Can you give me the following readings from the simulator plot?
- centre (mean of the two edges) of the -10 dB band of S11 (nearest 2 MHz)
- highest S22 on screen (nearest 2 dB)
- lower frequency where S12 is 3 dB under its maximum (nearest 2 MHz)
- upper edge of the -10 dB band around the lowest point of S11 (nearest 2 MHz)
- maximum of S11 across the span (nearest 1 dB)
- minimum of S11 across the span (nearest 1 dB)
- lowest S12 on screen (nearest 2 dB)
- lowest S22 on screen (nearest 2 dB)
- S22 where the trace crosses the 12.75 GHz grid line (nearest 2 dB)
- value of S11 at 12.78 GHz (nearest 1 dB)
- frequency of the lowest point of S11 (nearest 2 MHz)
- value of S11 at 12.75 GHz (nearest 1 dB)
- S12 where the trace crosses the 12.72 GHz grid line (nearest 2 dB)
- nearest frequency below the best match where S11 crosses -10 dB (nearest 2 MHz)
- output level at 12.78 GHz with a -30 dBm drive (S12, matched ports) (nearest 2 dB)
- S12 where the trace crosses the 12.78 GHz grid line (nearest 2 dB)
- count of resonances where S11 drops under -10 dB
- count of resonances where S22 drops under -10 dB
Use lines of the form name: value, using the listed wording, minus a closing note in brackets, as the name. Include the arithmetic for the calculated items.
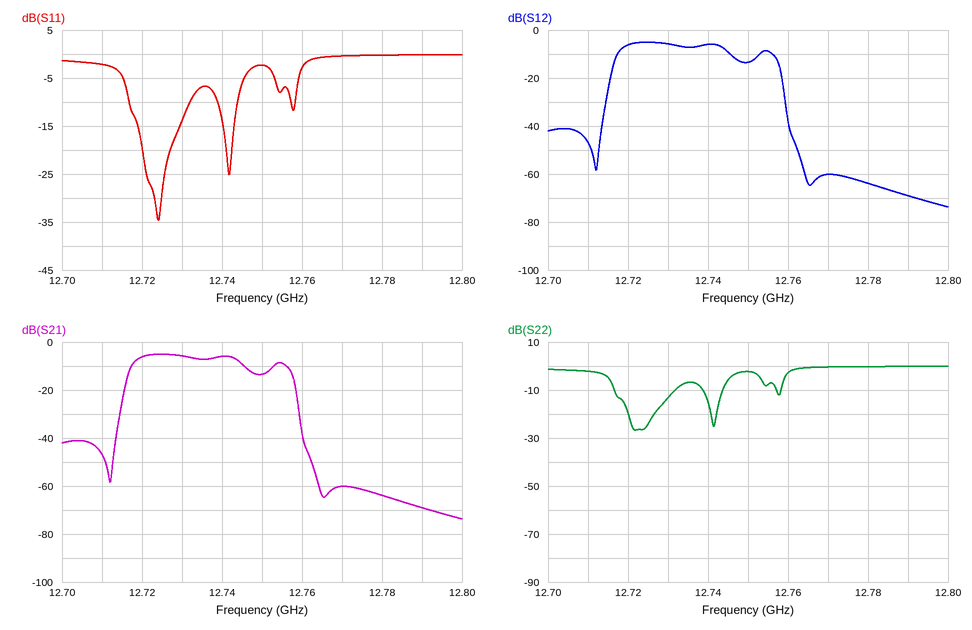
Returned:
centre (mean of the two edges) of the -10 dB band of S11: 12.724 GHz
highest S22 on screen: 0 dB
lower frequency where S12 is 3 dB under its maximum: 12.718 GHz
upper edge of the -10 dB band around the lowest point of S11: 12.732 GHz
maximum of S11 across the span: 0 dB
minimum of S11 across the span: -35 dB
lowest S12 on screen: -74 dB
lowest S22 on screen: -26 dB
S22 where the trace crosses the 12.75 GHz grid line: -2 dB
value of S11 at 12.78 GHz: 0 dB
frequency of the lowest point of S11: 12.724 GHz
value of S11 at 12.75 GHz: -2 dB
S12 where the trace crosses the 12.72 GHz grid line: -6 dB
nearest frequency below the best match where S11 crosses -10 dB: 12.716 GHz
output level at 12.78 GHz with a -30 dBm drive (S12, matched ports): -30 dBm + (-64 dB) = -94 dBm
S12 where the trace crosses the 12.78 GHz grid line: -64 dB
count of resonances where S11 drops under -10 dB: 3
count of resonances where S22 drops under -10 dB: 3
